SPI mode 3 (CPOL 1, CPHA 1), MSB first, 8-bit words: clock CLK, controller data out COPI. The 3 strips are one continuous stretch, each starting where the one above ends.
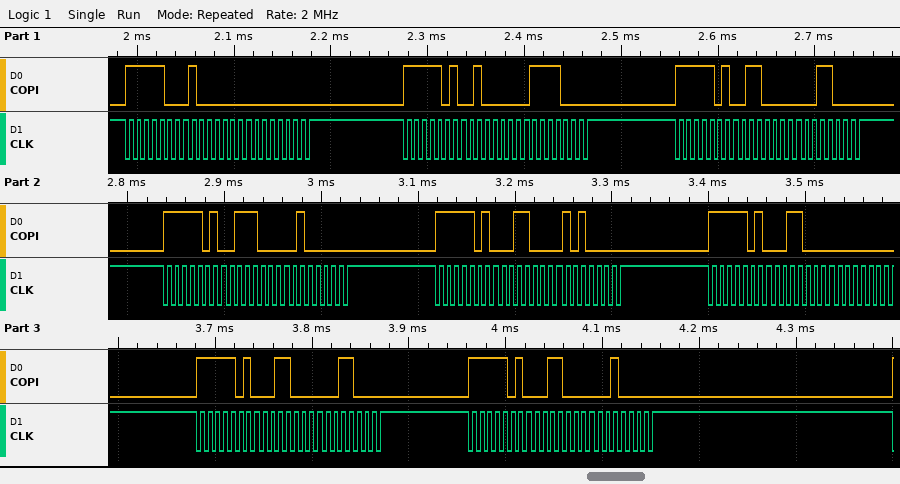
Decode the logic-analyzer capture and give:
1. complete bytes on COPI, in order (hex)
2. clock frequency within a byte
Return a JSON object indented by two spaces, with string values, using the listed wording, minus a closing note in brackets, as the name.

{
  "complete bytes on COPI, in order": "F8 80 00 FA 40 F0 FA 60 30 FA 70 40 FA 30 A0 FA 30 00 FA 30 30 FA 30 20",
  "clock frequency within a byte": "125 kHz"
}
